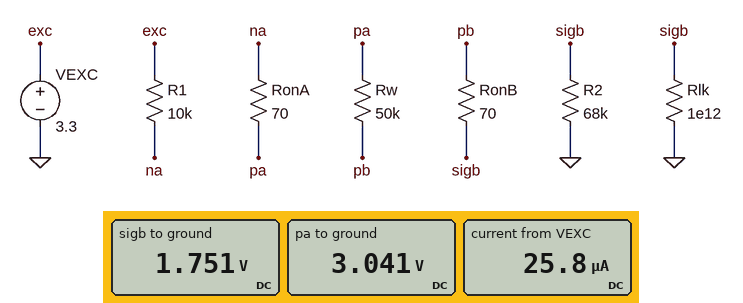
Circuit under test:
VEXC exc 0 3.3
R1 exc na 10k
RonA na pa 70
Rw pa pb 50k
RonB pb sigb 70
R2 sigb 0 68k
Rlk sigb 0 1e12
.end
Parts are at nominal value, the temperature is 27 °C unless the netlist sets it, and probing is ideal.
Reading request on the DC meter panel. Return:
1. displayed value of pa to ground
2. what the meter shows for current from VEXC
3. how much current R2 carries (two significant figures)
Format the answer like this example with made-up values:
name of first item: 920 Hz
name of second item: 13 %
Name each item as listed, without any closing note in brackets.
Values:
displayed value of pa to ground: 3.041 V
what the meter shows for current from VEXC: 25.8 µA
how much current R2 carries: 26 µA
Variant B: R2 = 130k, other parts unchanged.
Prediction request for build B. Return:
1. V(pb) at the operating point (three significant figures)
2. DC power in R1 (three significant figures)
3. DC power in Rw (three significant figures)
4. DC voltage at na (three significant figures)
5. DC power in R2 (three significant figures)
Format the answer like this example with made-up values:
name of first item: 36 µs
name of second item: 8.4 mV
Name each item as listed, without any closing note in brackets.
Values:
V(pb) at the operating point: 2.26 V
DC power in R1: 3.01 µW
DC power in Rw: 15.1 µW
DC voltage at na: 3.13 V
DC power in R2: 39.2 µW
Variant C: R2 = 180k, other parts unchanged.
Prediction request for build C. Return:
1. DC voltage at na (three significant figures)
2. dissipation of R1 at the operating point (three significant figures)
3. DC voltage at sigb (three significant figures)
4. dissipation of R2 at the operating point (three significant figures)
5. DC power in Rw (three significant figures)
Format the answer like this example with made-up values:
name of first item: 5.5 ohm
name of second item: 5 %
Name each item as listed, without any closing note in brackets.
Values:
DC voltage at na: 3.16 V
dissipation of R1 at the operating point: 1.89 µW
DC voltage at sigb: 2.47 V
dissipation of R2 at the operating point: 34.0 µW
DC power in Rw: 9.44 µW
